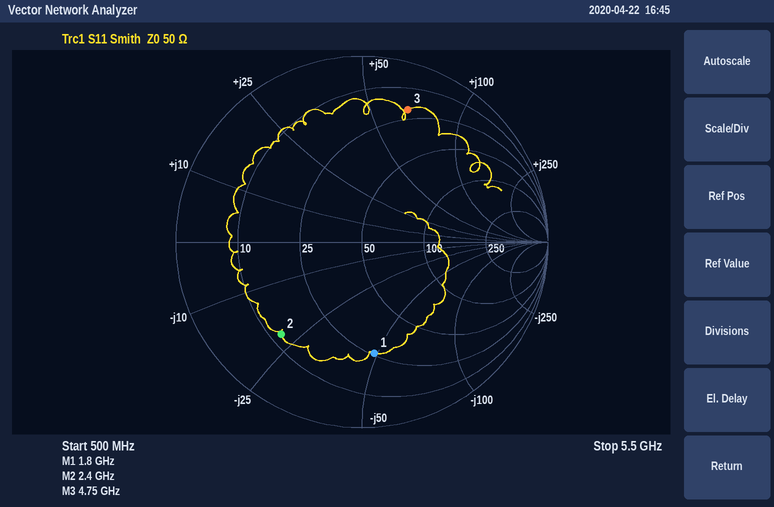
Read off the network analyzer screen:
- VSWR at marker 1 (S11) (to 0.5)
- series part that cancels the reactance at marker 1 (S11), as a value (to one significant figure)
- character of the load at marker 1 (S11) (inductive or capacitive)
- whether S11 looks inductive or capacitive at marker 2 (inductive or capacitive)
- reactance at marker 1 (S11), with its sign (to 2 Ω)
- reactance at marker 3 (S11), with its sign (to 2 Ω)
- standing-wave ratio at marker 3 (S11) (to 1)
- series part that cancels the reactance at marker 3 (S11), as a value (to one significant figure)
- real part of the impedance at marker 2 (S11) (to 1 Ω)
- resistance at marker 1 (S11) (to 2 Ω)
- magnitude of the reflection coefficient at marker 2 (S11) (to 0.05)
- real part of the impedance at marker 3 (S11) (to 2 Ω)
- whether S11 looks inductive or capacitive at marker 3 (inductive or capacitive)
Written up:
4.0
4 nH
capacitive
capacitive
-48 Ω
+66 Ω
7
500 fF
12 Ω
26 Ω
0.65
20 Ω
inductive
